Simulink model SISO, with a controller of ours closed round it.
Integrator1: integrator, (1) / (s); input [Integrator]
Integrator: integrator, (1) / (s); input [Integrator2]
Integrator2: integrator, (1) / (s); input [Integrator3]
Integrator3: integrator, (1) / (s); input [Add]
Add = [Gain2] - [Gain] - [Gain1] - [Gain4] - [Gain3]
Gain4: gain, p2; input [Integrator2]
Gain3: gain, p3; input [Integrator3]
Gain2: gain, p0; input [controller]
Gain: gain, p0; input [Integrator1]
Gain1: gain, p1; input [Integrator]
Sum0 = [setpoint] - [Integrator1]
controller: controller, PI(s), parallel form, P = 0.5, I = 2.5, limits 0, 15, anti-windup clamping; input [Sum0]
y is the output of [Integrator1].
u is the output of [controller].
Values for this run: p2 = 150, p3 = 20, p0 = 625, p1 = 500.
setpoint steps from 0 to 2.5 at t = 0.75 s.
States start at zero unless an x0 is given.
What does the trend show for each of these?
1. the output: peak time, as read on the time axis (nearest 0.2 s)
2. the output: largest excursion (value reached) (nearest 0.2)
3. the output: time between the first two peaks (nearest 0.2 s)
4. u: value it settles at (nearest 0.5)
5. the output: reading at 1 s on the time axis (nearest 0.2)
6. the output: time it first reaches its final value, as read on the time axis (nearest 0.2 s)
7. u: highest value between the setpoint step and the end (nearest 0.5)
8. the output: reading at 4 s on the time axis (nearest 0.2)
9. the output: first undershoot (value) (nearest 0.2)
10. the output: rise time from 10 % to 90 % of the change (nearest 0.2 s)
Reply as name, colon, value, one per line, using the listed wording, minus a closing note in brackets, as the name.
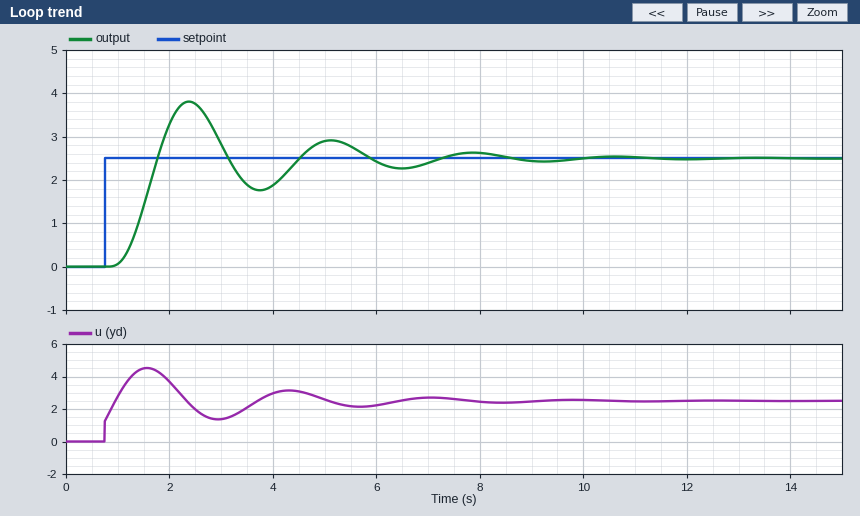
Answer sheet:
the output: peak time, as read on the time axis: 2.4 s
the output: largest excursion (value reached): 3.8
the output: time between the first two peaks: 2.8 s
u: value it settles at: 2.5
the output: reading at 1 s on the time axis: 0.0
the output: time it first reaches its final value, as read on the time axis: 1.8 s
u: highest value between the setpoint step and the end: 4.5
the output: reading at 4 s on the time axis: 1.8
the output: first undershoot (value): 1.8
the output: rise time from 10 % to 90 % of the change: 0.6 s
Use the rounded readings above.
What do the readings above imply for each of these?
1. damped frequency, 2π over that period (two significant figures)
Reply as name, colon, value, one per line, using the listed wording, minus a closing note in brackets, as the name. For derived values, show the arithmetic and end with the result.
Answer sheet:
damped frequency, 2π over that period: 2π / 2.8 = 2.2 rad/s
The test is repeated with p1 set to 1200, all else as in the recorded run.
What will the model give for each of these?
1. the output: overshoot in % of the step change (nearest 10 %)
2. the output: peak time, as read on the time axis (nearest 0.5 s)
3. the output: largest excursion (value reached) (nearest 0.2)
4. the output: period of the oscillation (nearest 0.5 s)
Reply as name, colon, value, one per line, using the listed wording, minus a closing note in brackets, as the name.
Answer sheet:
the output: overshoot in % of the step change: 40 %
the output: peak time, as read on the time axis: 3.5 s
the output: largest excursion (value reached): 3.6
the output: period of the oscillation: 5.5 s
